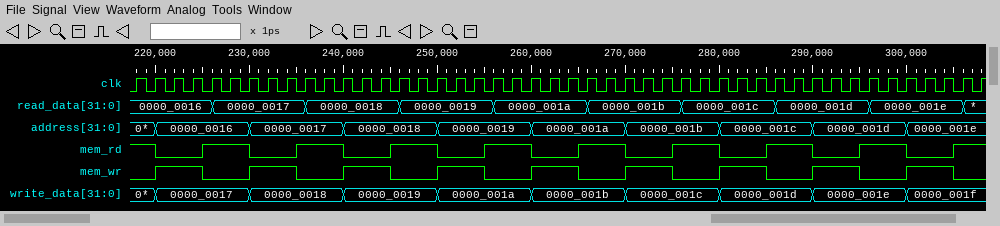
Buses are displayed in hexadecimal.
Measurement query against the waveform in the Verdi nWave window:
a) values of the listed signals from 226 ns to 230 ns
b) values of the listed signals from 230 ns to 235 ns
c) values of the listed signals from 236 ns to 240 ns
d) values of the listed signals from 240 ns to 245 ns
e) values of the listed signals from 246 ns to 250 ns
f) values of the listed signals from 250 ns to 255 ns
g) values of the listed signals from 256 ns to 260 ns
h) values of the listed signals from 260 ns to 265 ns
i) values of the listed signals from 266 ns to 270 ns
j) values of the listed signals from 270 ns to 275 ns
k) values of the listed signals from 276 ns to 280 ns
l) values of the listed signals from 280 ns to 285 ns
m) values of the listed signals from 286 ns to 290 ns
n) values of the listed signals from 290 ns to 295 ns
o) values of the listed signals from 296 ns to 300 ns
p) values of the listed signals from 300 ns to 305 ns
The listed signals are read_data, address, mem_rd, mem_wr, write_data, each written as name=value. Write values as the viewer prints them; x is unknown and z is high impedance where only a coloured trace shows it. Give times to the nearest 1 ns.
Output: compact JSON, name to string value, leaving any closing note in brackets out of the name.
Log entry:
{"values of the listed signals from 226 ns to 230 ns": "read_data=0000_0017, address=0000_0016, mem_rd=1, mem_wr=0, write_data=0000_0017", "values of the listed signals from 230 ns to 235 ns": "read_data=0000_0017, address=0000_0017, mem_rd=0, mem_wr=1, write_data=0000_0018", "values of the listed signals from 236 ns to 240 ns": "read_data=0000_0018, address=0000_0017, mem_rd=1, mem_wr=0, write_data=0000_0018", "values of the listed signals from 240 ns to 245 ns": "read_data=0000_0018, address=0000_0018, mem_rd=0, mem_wr=1, write_data=0000_0019", "values of the listed signals from 246 ns to 250 ns": "read_data=0000_0019, address=0000_0018, mem_rd=1, mem_wr=0, write_data=0000_0019", "values of the listed signals from 250 ns to 255 ns": "read_data=0000_0019, address=0000_0019, mem_rd=0, mem_wr=1, write_data=0000_001a", "values of the listed signals from 256 ns to 260 ns": "read_data=0000_001a, address=0000_0019, mem_rd=1, mem_wr=0, write_data=0000_001a", "values of the listed signals from 260 ns to 265 ns": "read_data=0000_001a, address=0000_001a, mem_rd=0, mem_wr=1, write_data=0000_001b", "values of the listed signals from 266 ns to 270 ns": "read_data=0000_001b, address=0000_001a, mem_rd=1, mem_wr=0, write_data=0000_001b", "values of the listed signals from 270 ns to 275 ns": "read_data=0000_001b, address=0000_001b, mem_rd=0, mem_wr=1, write_data=0000_001c", "values of the listed signals from 276 ns to 280 ns": "read_data=0000_001c, address=0000_001b, mem_rd=1, mem_wr=0, write_data=0000_001c", "values of the listed signals from 280 ns to 285 ns": "read_data=0000_001c, address=0000_001c, mem_rd=0, mem_wr=1, write_data=0000_001d", "values of the listed signals from 286 ns to 290 ns": "read_data=0000_001d, address=0000_001c, mem_rd=1, mem_wr=0, write_data=0000_001d", "values of the listed signals from 290 ns to 295 ns": "read_data=0000_001d, address=0000_001d, mem_rd=0, mem_wr=1, write_data=0000_001e", "values of the listed signals from 296 ns to 300 ns": "read_data=0000_001e, address=0000_001d, mem_rd=1, mem_wr=0, write_data=0000_001e", "values of the listed signals from 300 ns to 305 ns": "read_data=0000_001e, address=0000_001e, mem_rd=0, mem_wr=1, write_data=0000_001f"}
